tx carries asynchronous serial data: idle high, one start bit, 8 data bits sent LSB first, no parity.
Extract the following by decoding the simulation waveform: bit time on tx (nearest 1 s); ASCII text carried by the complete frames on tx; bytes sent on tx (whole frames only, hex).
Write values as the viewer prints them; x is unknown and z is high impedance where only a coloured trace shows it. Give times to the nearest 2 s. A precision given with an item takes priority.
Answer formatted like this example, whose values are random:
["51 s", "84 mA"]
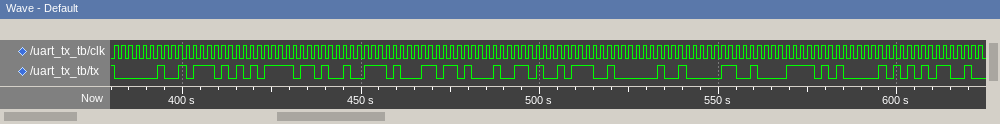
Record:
["2 s", "\" World: 0xA5\"", "20, 57, 6F, 72, 6C, 64, 3A, 20, 30, 78, 41, 35"]
